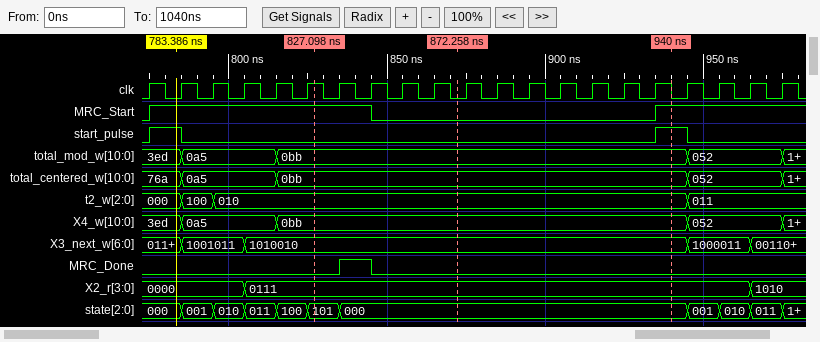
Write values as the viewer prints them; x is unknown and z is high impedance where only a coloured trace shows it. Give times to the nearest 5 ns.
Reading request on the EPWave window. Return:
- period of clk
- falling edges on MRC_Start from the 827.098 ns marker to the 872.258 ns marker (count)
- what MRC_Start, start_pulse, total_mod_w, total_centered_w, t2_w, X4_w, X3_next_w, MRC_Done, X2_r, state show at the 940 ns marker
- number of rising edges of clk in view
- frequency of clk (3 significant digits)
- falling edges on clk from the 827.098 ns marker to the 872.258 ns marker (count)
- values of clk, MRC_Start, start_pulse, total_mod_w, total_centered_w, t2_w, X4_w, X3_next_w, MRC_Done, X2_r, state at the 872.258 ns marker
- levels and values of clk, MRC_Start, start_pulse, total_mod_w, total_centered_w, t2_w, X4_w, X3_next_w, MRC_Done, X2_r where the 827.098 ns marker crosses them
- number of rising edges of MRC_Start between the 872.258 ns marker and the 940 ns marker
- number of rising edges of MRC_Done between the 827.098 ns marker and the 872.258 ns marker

10 ns
1
MRC_Start=1, start_pulse=1, total_mod_w=0bb, total_centered_w=0bb, t2_w=010, X4_w=0bb, X3_next_w=1010010, MRC_Done=0, X2_r=0111, state=000
21
100 MHz
5
clk=0, MRC_Start=0, start_pulse=0, total_mod_w=0bb, total_centered_w=0bb, t2_w=010, X4_w=0bb, X3_next_w=1010010, MRC_Done=0, X2_r=0111, state=000
clk=1, MRC_Start=1, start_pulse=0, total_mod_w=0bb, total_centered_w=0bb, t2_w=010, X4_w=0bb, X3_next_w=1010010, MRC_Done=0, X2_r=0111
1
1
